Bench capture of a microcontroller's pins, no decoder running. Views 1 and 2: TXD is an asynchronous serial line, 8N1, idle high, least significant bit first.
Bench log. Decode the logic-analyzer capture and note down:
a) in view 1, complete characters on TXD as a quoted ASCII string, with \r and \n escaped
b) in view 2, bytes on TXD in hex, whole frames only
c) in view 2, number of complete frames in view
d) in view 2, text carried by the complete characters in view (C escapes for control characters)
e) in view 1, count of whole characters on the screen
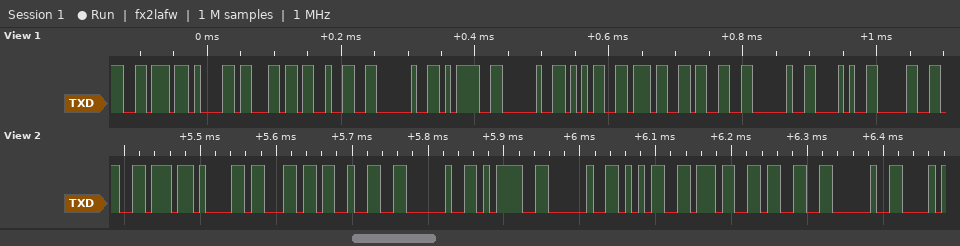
"val2 = 573 (0"
0x76 0x61 0x6C 0x32 0x20 0x3D 0x20 0x35 0x37 0x33 0x20
11
"val2 = 573 "
13
